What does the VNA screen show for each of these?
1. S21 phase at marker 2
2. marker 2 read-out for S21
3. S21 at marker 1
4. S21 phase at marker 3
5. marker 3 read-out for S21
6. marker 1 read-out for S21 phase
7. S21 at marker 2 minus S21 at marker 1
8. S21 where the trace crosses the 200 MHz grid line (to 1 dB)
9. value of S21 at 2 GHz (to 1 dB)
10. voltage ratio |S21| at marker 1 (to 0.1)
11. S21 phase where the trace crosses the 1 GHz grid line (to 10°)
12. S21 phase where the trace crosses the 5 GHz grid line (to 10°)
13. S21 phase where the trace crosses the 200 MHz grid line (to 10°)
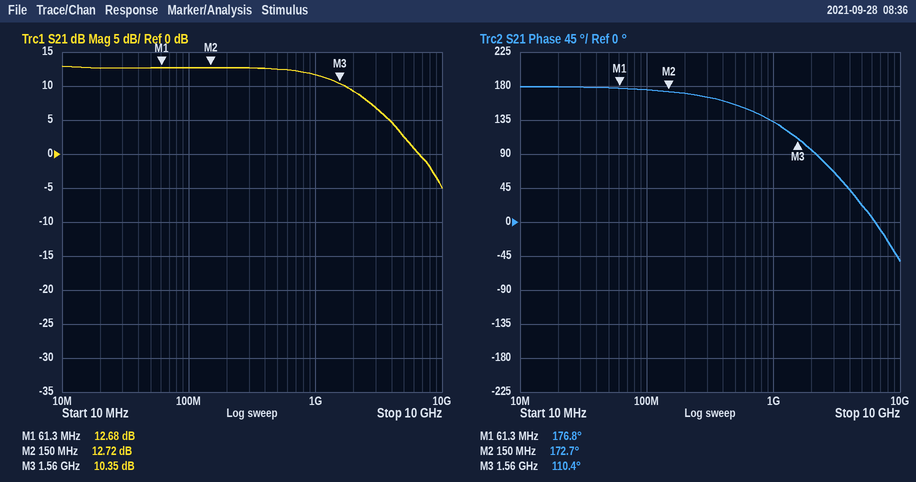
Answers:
172.7°
12.72 dB
12.68 dB
110.4°
10.35 dB
176.8°
0.04 dB
13 dB
9 dB
4.3
130°
20°
170°
